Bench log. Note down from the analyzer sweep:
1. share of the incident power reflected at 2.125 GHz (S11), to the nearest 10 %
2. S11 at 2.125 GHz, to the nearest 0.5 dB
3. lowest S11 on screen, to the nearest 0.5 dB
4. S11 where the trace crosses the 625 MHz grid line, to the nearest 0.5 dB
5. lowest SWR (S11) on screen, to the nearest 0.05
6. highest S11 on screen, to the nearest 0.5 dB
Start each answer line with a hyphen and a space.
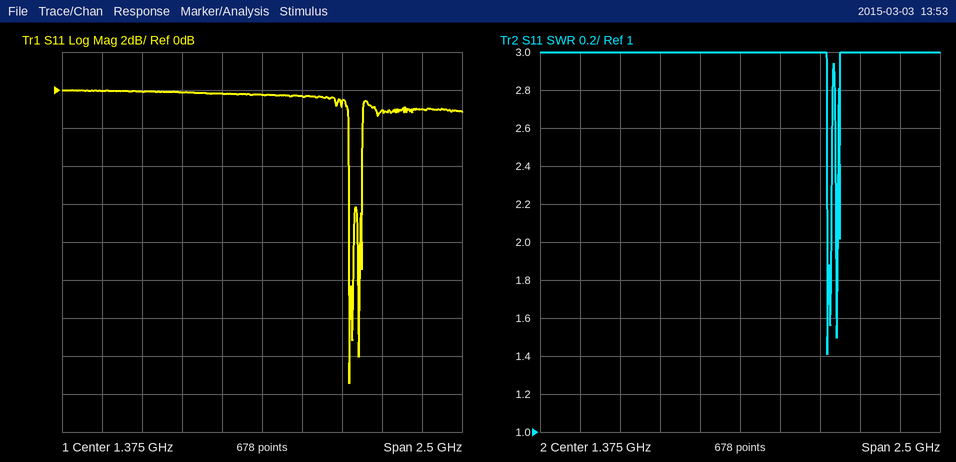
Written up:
- 80 %
- -1.0 dB
- -15.5 dB
- 0.0 dB
- 1.40
- 0.0 dB
